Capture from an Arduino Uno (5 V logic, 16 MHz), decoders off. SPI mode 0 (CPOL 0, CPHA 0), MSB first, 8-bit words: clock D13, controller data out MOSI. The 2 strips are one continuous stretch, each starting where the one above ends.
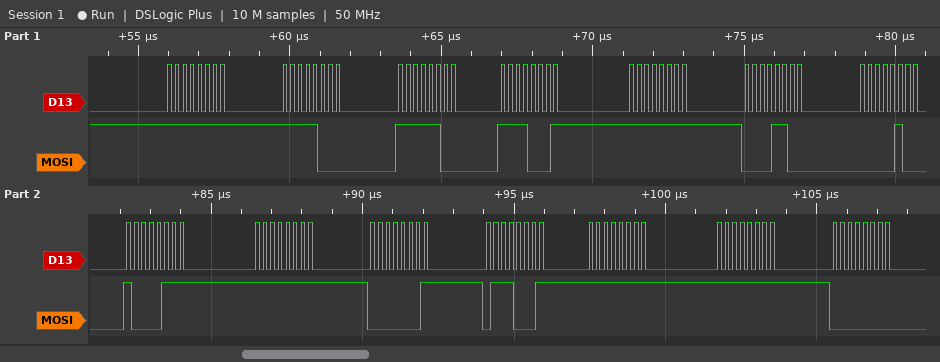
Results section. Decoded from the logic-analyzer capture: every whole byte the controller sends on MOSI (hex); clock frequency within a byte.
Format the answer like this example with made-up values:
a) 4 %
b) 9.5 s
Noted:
a) FF F8 FC F1 FF 0C 04 87 FF 01 71 FF FF 00
b) 4 MHz
